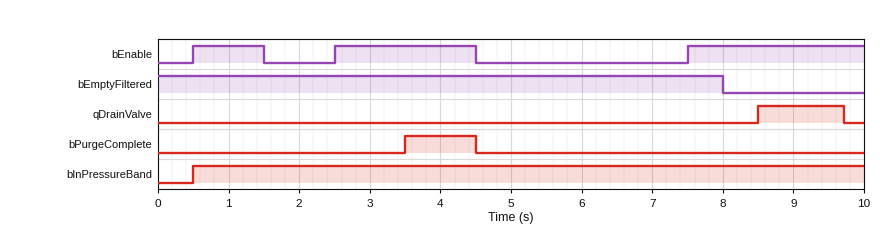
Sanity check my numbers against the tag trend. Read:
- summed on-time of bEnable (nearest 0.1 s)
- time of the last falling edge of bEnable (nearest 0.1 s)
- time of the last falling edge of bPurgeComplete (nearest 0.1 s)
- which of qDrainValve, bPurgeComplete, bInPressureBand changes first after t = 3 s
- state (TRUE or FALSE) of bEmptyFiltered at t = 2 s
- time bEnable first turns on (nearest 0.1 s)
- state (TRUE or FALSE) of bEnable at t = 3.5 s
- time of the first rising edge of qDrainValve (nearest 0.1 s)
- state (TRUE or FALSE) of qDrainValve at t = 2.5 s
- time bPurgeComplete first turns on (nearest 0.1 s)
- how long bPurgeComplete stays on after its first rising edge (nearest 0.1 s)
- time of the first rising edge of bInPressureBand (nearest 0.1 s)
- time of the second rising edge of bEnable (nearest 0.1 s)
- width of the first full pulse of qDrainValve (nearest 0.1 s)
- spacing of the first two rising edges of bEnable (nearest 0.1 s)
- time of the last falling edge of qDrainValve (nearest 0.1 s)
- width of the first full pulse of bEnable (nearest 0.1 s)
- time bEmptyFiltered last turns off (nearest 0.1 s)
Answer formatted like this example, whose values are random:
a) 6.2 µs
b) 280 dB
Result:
a) 5.5 s
b) 4.5 s
c) 4.5 s
d) bPurgeComplete
e) TRUE
f) 0.5 s
g) TRUE
h) 8.5 s
i) FALSE
j) 3.5 s
k) 1.0 s
l) 0.5 s
m) 2.5 s
n) 1.2 s
o) 2.0 s
p) 9.7 s
q) 1.0 s
r) 8.0 s
